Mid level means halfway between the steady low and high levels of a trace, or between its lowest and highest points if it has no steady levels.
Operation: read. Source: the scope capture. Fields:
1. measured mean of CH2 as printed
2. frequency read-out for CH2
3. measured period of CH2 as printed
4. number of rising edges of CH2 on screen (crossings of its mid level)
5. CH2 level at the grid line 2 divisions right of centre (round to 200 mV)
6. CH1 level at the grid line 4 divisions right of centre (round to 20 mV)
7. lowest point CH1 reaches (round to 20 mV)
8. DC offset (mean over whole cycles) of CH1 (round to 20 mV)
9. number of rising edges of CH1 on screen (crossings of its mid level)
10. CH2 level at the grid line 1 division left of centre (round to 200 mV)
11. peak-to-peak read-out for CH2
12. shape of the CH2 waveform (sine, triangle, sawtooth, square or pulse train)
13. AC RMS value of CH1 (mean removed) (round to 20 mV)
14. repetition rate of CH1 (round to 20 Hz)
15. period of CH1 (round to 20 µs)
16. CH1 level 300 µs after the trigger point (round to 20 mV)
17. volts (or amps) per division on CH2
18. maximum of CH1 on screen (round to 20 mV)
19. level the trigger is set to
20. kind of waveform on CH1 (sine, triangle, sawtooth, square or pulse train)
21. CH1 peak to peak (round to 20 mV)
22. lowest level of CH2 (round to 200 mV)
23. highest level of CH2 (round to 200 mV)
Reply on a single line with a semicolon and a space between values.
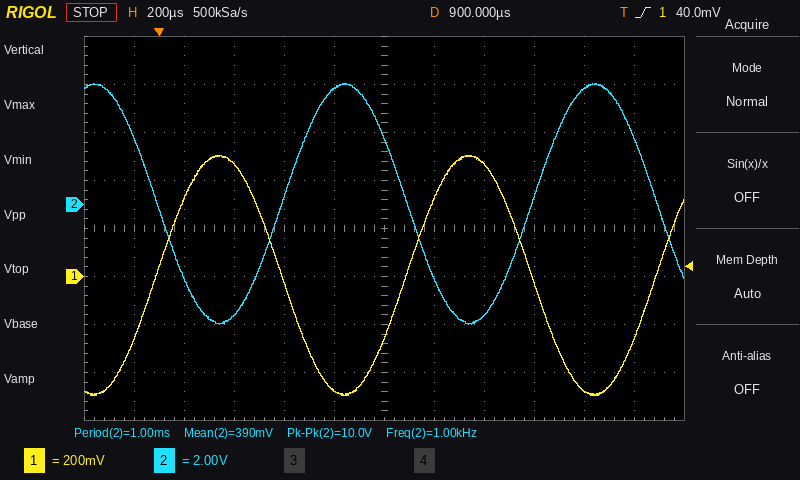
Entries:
390 mV; 1.00 kHz; 1.00 ms; 2; -4.6 V; -480 mV; -500 mV; 0 mV; 3; 4.8 V; 10.0 V; sine; 360 mV; 1.00 kHz; 1.00 ms; 460 mV; 2 V; 500 mV; 40.0 mV; sine; 1.00 V; -5.0 V; 5.0 V
